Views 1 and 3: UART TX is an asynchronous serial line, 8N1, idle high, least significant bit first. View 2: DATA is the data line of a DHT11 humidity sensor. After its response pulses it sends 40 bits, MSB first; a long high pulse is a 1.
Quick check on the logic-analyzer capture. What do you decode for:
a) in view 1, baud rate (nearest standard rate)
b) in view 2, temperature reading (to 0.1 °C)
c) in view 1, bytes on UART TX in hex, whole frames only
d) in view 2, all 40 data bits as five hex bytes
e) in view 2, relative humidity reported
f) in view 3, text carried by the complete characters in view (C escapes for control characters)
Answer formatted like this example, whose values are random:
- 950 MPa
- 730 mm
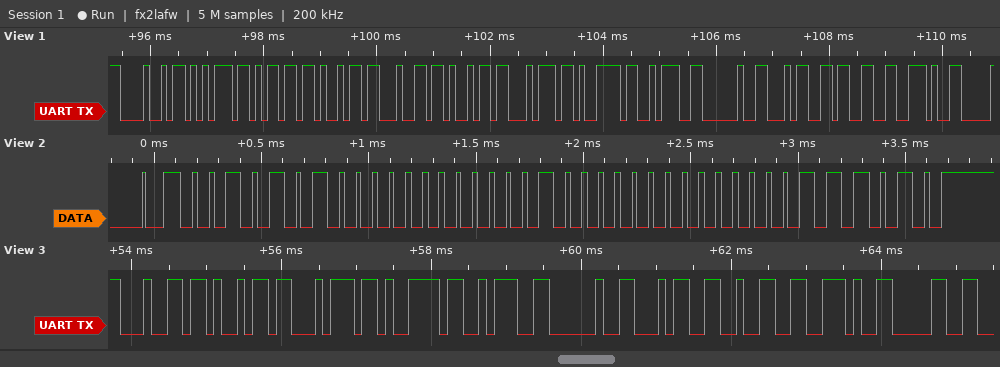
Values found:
- 9600 baud
- 16.0 °C
- 48 75 6D 69 64 69 74 79 3A 20 34 33 2E
- 2A 00 10 00 3A
- 42 %
- "dity: 42.0"
